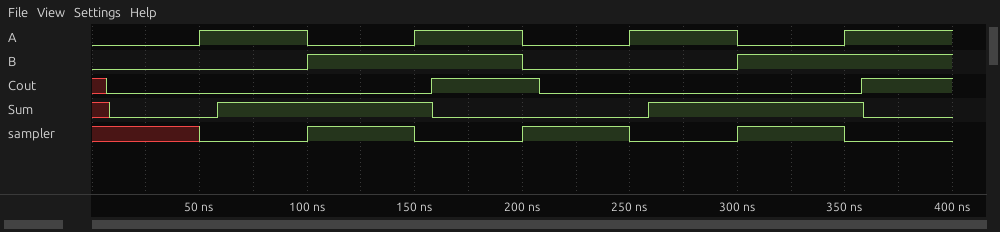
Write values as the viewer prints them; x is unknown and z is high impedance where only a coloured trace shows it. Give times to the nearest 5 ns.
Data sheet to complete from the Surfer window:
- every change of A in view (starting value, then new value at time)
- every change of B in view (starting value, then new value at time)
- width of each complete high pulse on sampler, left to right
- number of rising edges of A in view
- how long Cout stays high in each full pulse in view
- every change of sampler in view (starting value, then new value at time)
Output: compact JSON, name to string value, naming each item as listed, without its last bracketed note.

{"every change of A in view": "0, 1 at 50 ns, 0 at 100 ns, 1 at 150 ns, 0 at 200 ns, 1 at 250 ns, 0 at 300 ns, 1 at 350 ns", "every change of B in view": "0, 1 at 100 ns, 0 at 200 ns, 1 at 300 ns", "width of each complete high pulse on sampler, left to right": "50 ns, 50 ns, 50 ns", "number of rising edges of A in view": "4", "how long Cout stays high in each full pulse in view": "50 ns", "every change of sampler in view": "x, 0 at 50 ns, 1 at 100 ns, 0 at 150 ns, 1 at 200 ns, 0 at 250 ns, 1 at 300 ns, 0 at 350 ns"}
